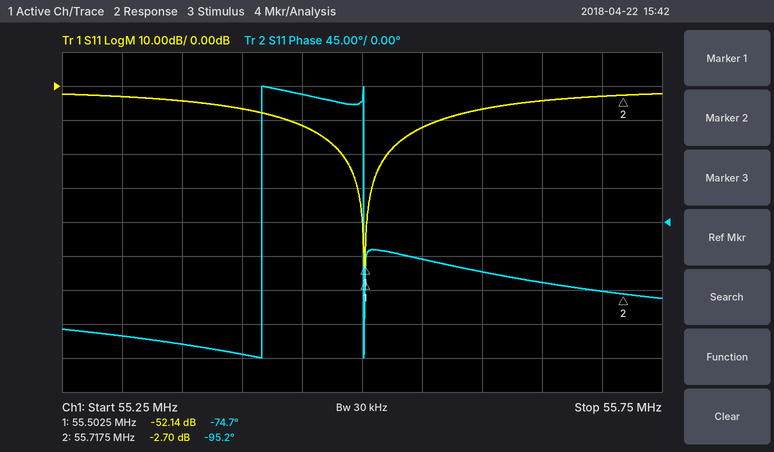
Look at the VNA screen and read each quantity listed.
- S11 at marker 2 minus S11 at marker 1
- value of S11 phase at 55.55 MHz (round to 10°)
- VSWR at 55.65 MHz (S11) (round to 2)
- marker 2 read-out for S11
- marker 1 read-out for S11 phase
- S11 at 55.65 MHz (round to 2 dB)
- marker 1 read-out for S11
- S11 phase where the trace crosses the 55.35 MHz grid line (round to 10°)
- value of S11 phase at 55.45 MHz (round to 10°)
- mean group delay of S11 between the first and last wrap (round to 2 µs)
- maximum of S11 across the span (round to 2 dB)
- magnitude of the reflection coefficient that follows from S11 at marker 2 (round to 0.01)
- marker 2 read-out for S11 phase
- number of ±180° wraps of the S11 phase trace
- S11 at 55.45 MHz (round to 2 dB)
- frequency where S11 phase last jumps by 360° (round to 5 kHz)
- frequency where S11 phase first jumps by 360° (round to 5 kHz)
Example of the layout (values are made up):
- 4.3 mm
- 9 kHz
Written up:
- 49.44 dB
- -50°
- 4
- -2.70 dB
- -74.7°
- -4 dB
- -52.14 dB
- -160°
- 170°
- 12 µs
- -2 dB
- 0.73
- -95.2°
- 2
- -12 dB
- 55.500 MHz
- 55.415 MHz
